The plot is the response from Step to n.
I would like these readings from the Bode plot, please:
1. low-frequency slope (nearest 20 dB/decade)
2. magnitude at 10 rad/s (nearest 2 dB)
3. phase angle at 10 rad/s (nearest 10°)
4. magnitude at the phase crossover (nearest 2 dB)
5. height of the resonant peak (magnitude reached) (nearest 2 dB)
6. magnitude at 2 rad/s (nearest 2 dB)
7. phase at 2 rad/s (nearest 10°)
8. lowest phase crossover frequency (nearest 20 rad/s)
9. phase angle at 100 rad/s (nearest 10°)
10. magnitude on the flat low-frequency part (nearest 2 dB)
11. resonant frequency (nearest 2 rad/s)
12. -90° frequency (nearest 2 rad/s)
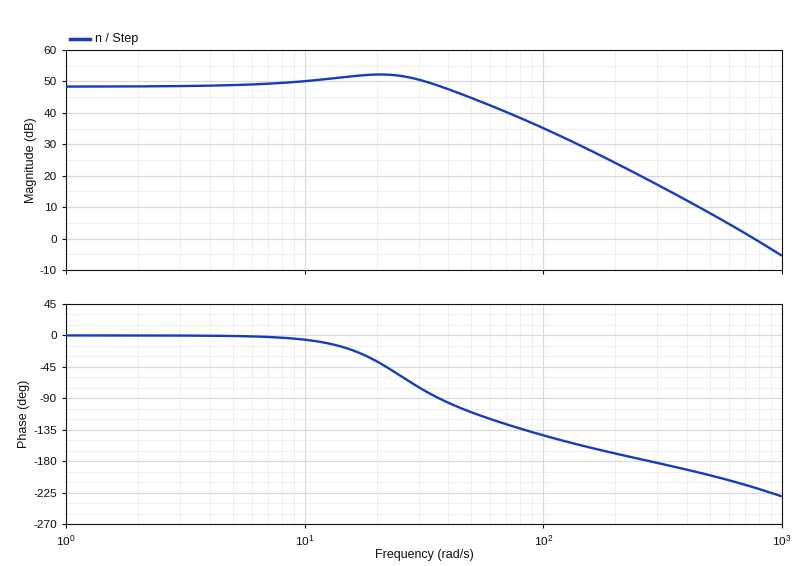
0 dB/decade
50 dB
-10°
18 dB
52 dB
48 dB
0°
280 rad/s
-140°
48 dB
20 rad/s
36 rad/s
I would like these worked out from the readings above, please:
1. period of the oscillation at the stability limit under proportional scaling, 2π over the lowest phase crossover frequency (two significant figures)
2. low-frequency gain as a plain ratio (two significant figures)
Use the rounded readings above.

0.022 s
250
